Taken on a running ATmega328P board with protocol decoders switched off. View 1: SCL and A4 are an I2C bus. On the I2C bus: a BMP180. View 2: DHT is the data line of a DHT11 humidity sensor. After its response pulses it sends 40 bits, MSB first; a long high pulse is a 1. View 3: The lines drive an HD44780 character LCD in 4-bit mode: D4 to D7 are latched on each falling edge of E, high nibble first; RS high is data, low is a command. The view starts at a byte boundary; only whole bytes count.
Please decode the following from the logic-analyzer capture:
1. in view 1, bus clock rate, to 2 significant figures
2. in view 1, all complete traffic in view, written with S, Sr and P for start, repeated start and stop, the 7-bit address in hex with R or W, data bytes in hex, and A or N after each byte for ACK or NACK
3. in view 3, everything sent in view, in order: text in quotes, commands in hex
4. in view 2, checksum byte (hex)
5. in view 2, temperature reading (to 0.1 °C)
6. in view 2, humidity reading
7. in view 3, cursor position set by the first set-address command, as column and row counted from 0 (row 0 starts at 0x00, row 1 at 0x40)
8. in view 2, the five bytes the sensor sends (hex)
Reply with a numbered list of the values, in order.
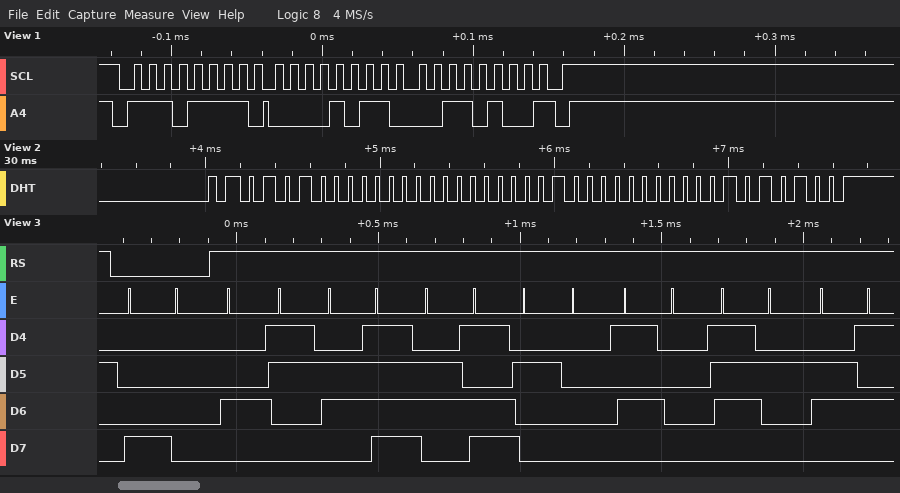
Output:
1. 100 kHz
2. S 77R A 0B A 34 N P
3. 0x80 "Com Pre"
4. 0x54
5. 4.0 °C
6. 80 %
7. column 0, row 0
8. 50 00 04 00 54
